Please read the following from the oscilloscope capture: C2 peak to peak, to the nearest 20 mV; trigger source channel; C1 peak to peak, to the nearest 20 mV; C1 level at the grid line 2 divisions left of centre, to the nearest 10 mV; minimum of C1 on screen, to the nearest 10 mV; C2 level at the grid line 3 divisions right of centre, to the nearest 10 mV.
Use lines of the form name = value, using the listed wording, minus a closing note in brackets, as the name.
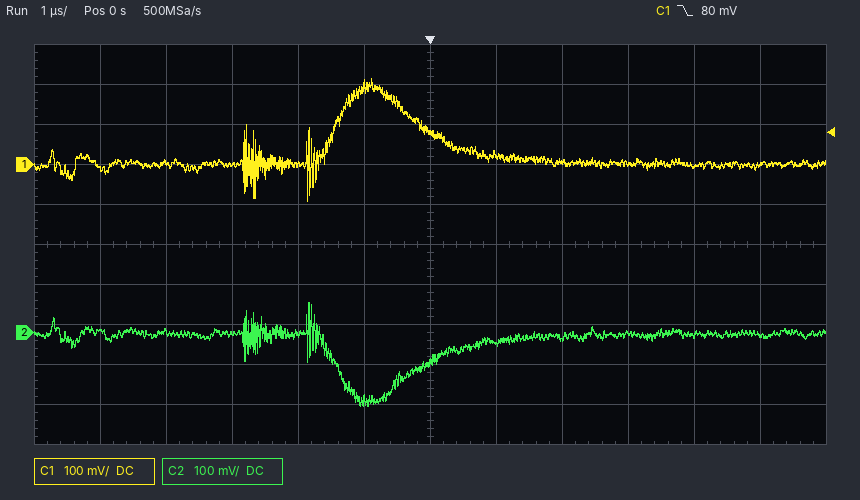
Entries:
C2 peak to peak, to the nearest 20 mV = 260 mV
trigger source channel = C1
C1 peak to peak, to the nearest 20 mV = 300 mV
C1 level at the grid line 2 divisions left of centre, to the nearest 10 mV = 0 mV
minimum of C1 on screen, to the nearest 10 mV = -90 mV
C2 level at the grid line 3 divisions right of centre, to the nearest 10 mV = 0 mV
